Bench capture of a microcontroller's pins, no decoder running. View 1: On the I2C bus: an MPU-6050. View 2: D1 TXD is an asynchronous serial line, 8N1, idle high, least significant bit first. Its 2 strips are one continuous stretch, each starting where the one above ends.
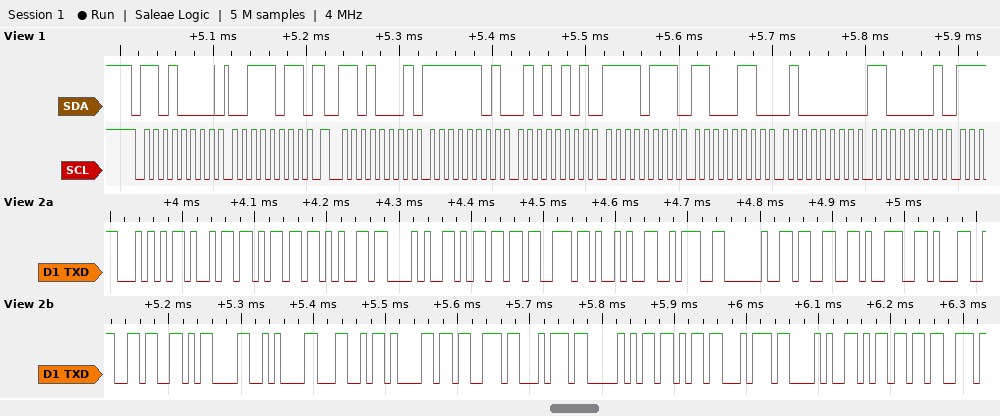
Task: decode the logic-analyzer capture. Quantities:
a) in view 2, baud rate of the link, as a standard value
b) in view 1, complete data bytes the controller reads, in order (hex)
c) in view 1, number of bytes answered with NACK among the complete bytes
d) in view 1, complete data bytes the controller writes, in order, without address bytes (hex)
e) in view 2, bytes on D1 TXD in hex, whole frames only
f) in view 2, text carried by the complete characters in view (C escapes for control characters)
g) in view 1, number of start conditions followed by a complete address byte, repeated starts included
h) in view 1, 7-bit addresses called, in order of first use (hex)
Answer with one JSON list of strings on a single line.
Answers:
["115200 baud", "FD 55 F7 C6 40 C1", "0", "3B", "54 69 6D 65 28 6D 73 29 3A 20 33 39 31 36 0D 0A 4C 61 73 74 50 6B 74 28 6D 73", "\"Time(ms): 3916\\r\\nLastPkt(ms\"", "2", "0x68"]
